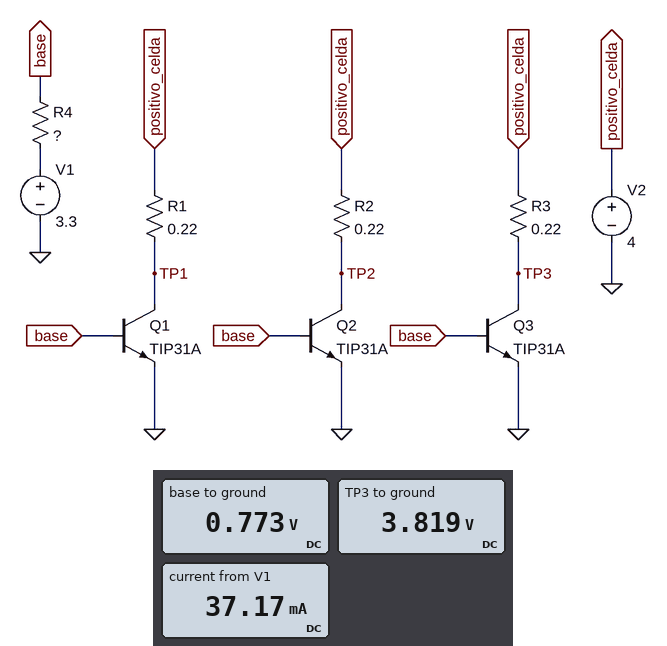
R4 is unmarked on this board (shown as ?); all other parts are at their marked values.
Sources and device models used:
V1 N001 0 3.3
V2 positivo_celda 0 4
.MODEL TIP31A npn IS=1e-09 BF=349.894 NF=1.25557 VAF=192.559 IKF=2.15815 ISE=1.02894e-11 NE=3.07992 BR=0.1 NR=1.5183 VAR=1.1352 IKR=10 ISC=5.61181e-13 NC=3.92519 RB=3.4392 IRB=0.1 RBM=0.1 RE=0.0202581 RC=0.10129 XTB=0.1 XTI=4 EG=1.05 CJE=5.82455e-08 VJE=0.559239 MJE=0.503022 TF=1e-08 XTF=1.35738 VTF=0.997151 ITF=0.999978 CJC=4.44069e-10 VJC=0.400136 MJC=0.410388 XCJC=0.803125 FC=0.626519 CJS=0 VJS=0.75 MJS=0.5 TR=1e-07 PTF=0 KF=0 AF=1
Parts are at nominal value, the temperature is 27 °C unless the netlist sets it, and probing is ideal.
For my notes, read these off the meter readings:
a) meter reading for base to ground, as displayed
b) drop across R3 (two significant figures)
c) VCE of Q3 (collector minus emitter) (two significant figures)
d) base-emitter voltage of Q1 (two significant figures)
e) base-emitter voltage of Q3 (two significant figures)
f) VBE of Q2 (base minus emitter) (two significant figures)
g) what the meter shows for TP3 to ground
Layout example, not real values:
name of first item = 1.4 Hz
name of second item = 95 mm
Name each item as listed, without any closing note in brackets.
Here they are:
meter reading for base to ground, as displayed = 0.773 V
drop across R3 = 180 mV
VCE of Q3 (collector minus emitter) = 3.8 V
base-emitter voltage of Q1 = 770 mV
base-emitter voltage of Q3 = 770 mV
VBE of Q2 (base minus emitter) = 770 mV
what the meter shows for TP3 to ground = 3.819 V
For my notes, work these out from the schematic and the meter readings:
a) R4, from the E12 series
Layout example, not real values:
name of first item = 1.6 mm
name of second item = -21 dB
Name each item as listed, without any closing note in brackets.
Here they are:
R4, from the E12 series = 68 Ω
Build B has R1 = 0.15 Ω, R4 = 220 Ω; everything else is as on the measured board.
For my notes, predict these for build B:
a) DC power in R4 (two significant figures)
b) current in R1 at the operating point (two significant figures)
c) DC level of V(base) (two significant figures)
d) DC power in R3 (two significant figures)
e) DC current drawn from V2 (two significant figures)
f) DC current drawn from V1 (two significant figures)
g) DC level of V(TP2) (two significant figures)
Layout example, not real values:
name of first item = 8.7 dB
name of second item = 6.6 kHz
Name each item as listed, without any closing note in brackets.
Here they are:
DC power in R4 = 31 mW
current in R1 at the operating point = 400 mA
DC level of V(base) = 700 mV
DC power in R3 = 34 mW
DC current drawn from V2 = 1.2 A
DC current drawn from V1 = 12 mA
DC level of V(TP2) = 3.9 V
